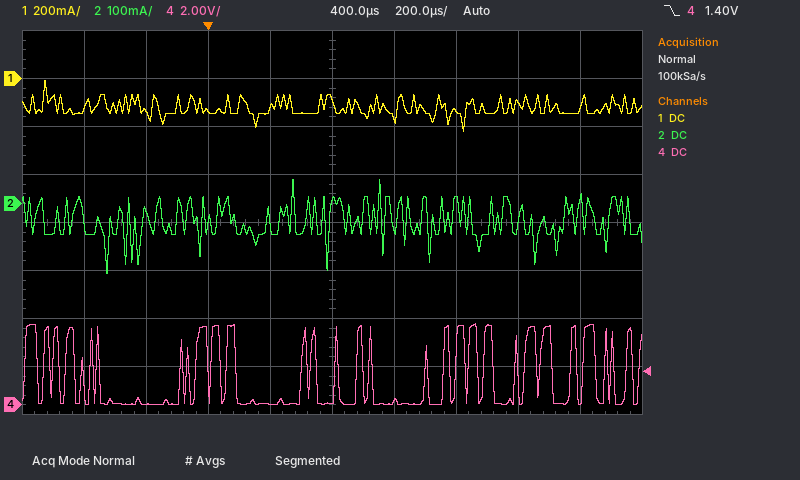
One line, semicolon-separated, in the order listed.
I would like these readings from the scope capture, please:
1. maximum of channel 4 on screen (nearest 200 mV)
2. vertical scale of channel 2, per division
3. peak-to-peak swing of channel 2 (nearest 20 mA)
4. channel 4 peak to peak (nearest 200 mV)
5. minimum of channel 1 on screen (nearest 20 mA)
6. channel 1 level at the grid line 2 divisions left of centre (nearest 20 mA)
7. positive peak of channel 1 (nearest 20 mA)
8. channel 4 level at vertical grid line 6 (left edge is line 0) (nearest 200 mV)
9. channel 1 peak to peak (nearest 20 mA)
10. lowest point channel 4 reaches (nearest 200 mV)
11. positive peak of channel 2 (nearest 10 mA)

3.4 V; 100 mA; 200 mA; 3.4 V; -220 mA; -140 mA; 0 mA; 200 mV; 220 mA; 0.0 V; 50 mA
